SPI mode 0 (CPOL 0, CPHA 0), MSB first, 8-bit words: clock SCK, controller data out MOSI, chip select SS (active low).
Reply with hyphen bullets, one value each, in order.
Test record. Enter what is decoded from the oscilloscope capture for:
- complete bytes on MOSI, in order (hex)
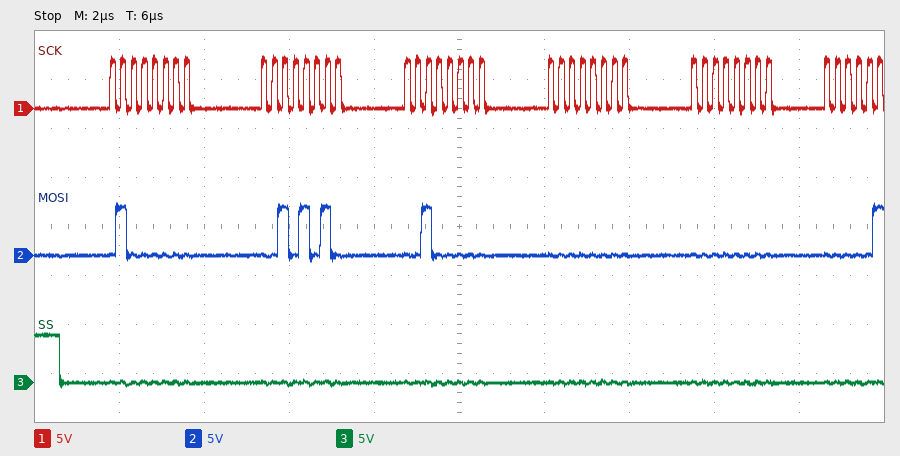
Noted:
- 40 2A 20 00 00
